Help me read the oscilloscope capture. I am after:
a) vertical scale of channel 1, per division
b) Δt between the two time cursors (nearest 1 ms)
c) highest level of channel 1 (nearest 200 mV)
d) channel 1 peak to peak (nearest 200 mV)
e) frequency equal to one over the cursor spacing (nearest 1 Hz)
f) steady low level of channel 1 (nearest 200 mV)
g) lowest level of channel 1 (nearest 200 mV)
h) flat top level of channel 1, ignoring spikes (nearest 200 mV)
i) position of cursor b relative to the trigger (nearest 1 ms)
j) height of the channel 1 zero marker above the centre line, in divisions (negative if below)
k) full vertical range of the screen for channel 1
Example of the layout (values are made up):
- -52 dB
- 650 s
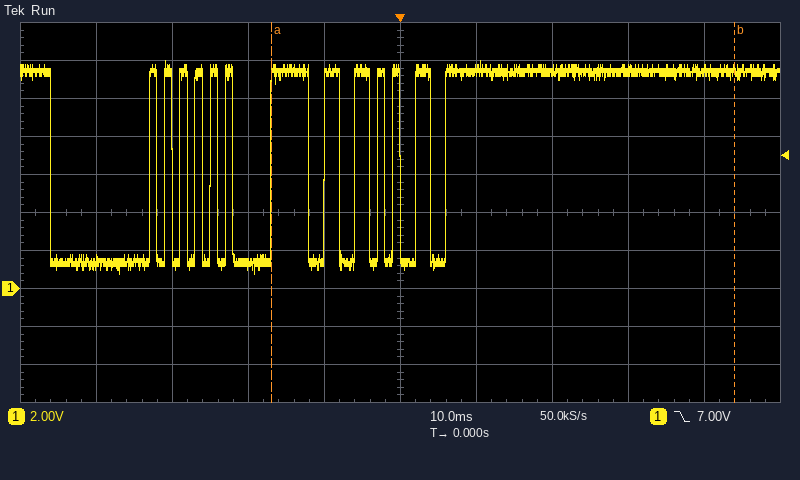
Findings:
- 2 V
- 61 ms
- 12.0 V
- 11.2 V
- 16 Hz
- 1.4 V
- 800 mV
- 11.4 V
- +44 ms
- -2.0 div
- 20 V
